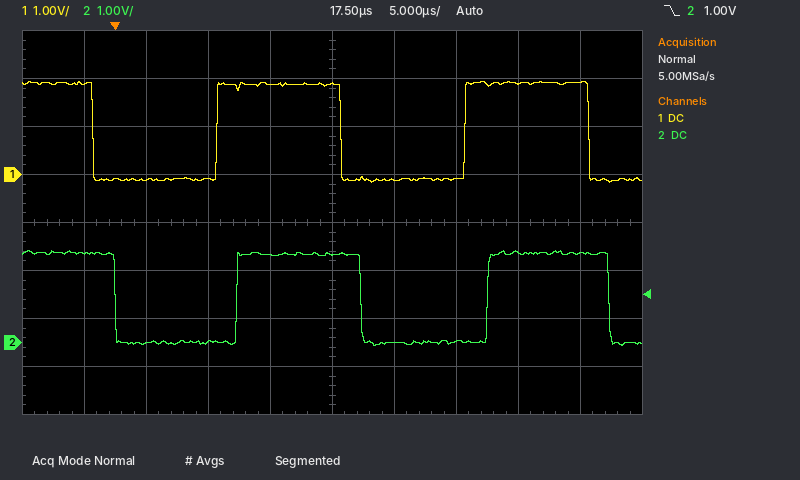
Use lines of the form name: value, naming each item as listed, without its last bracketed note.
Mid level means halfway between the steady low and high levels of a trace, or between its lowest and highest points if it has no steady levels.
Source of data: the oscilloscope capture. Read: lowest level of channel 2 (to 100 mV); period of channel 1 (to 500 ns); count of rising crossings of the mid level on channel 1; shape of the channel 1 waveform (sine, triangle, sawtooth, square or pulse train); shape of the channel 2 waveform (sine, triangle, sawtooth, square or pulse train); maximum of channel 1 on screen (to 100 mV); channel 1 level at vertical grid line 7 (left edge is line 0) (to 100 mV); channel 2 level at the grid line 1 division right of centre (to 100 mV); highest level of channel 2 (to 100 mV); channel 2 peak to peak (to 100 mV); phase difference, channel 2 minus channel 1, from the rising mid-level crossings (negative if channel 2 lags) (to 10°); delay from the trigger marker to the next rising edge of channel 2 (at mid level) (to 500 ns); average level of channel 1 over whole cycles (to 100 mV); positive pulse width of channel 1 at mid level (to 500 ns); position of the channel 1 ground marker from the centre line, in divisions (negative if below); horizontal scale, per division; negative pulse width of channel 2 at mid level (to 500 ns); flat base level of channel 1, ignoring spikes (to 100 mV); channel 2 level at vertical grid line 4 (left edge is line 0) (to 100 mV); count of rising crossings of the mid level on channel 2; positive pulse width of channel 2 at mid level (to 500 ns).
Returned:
lowest level of channel 2: -100 mV
period of channel 1: 20.0 µs
count of rising crossings of the mid level on channel 1: 2
shape of the channel 1 waveform: square
shape of the channel 2 waveform: square
maximum of channel 1 on screen: 1.9 V
channel 1 level at vertical grid line 7 (left edge is line 0): -100 mV
channel 2 level at the grid line 1 division right of centre: 0.0 V
highest level of channel 2: 1.9 V
channel 2 peak to peak: 2.0 V
phase difference, channel 2 minus channel 1, from the rising mid-level crossings (negative if channel 2 lags): -30°
delay from the trigger marker to the next rising edge of channel 2 (at mid level): 10.0 µs
average level of channel 1 over whole cycles: 900 mV
positive pulse width of channel 1 at mid level: 10.0 µs
position of the channel 1 ground marker from the centre line, in divisions: +1.0 div
horizontal scale, per division: 5 µs
negative pulse width of channel 2 at mid level: 10.0 µs
flat base level of channel 1, ignoring spikes: -100 mV
channel 2 level at vertical grid line 4 (left edge is line 0): 1.8 V
count of rising crossings of the mid level on channel 2: 2
positive pulse width of channel 2 at mid level: 10.0 µs
